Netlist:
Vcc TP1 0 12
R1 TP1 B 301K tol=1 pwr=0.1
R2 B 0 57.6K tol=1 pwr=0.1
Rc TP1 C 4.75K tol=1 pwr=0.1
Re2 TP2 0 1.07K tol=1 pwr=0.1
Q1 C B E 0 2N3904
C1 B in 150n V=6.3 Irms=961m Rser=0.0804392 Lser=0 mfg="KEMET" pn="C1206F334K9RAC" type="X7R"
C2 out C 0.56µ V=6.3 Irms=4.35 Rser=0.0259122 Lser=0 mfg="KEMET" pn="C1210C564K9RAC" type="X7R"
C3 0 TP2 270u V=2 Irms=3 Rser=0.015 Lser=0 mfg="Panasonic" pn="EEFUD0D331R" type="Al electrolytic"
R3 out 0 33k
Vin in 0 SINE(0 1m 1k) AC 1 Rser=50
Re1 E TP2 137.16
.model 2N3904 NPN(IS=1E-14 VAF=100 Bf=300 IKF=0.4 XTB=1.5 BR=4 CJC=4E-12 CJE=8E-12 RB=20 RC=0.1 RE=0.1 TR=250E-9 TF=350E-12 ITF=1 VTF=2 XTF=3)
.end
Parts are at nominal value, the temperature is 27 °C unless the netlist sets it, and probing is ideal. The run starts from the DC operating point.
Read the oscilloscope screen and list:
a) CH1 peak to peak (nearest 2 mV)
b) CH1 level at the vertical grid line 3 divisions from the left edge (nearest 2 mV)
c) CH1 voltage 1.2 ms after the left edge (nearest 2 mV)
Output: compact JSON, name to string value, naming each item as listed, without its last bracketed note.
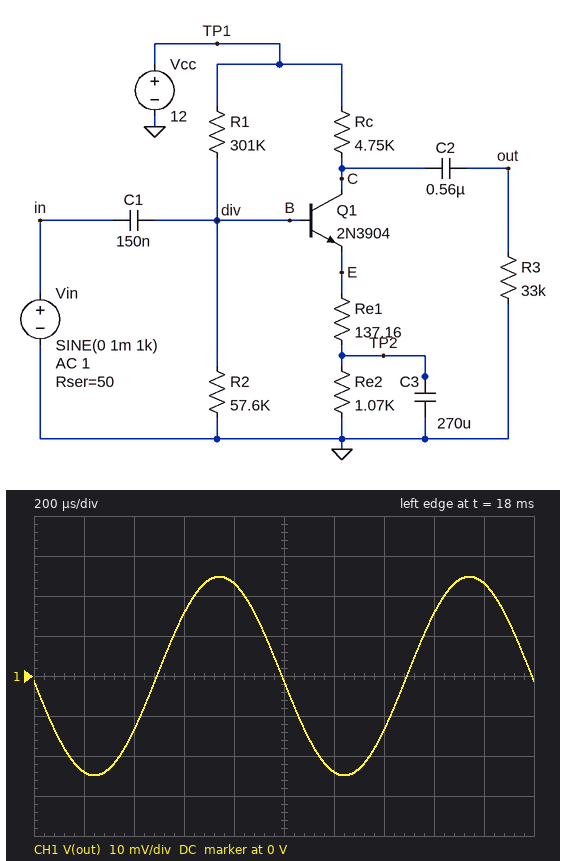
{"CH1 peak to peak": "50 mV", "CH1 level at the vertical grid line 3 divisions from the left edge": "16 mV", "CH1 voltage 1.2 ms after the left edge": "-24 mV"}
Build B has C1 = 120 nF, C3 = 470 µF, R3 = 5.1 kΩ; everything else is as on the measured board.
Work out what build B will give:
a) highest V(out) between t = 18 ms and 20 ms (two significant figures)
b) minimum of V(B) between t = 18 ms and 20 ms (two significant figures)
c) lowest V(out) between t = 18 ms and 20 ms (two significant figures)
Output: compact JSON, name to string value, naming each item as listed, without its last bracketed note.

{"highest V(out) between t = 18 ms and 20 ms": "15 mV", "minimum of V(B) between t = 18 ms and 20 ms": "1.8 V", "lowest V(out) between t = 18 ms and 20 ms": "-15 mV"}
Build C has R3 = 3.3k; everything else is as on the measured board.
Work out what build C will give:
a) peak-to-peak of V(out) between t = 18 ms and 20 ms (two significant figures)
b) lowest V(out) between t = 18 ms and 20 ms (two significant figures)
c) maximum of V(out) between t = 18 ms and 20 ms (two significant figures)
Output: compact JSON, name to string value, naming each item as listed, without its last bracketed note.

{"peak-to-peak of V(out) between t = 18 ms and 20 ms": "23 mV", "lowest V(out) between t = 18 ms and 20 ms": "-12 mV", "maximum of V(out) between t = 18 ms and 20 ms": "12 mV"}
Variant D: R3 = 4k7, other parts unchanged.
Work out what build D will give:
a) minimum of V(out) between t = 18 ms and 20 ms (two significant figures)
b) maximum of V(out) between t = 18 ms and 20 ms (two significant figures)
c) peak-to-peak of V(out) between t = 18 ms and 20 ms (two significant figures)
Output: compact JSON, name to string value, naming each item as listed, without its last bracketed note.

{"minimum of V(out) between t = 18 ms and 20 ms": "-14 mV", "maximum of V(out) between t = 18 ms and 20 ms": "14 mV", "peak-to-peak of V(out) between t = 18 ms and 20 ms": "28 mV"}
